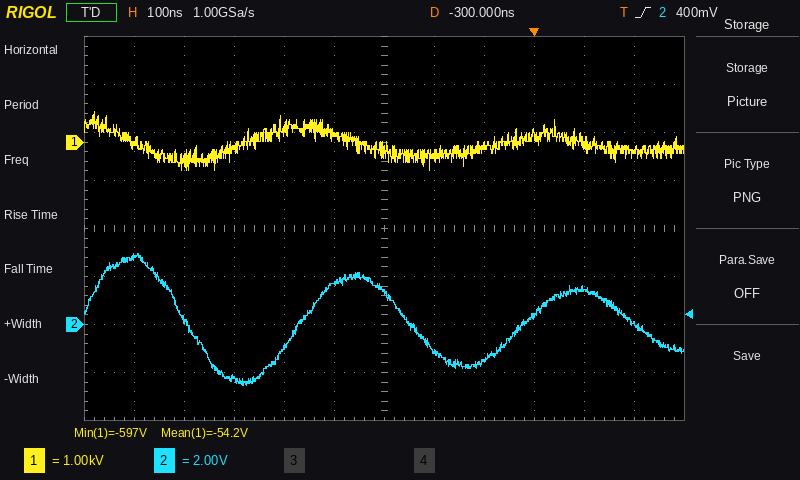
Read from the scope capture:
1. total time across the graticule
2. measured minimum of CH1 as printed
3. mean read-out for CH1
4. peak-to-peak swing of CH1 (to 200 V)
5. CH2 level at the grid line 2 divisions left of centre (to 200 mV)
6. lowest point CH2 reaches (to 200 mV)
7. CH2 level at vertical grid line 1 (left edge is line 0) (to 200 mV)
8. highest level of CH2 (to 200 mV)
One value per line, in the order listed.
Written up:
1.2 µs
-597 V
-54.2 V
1.2 kV
-1.0 V
-2.6 V
2.8 V
3.0 V
